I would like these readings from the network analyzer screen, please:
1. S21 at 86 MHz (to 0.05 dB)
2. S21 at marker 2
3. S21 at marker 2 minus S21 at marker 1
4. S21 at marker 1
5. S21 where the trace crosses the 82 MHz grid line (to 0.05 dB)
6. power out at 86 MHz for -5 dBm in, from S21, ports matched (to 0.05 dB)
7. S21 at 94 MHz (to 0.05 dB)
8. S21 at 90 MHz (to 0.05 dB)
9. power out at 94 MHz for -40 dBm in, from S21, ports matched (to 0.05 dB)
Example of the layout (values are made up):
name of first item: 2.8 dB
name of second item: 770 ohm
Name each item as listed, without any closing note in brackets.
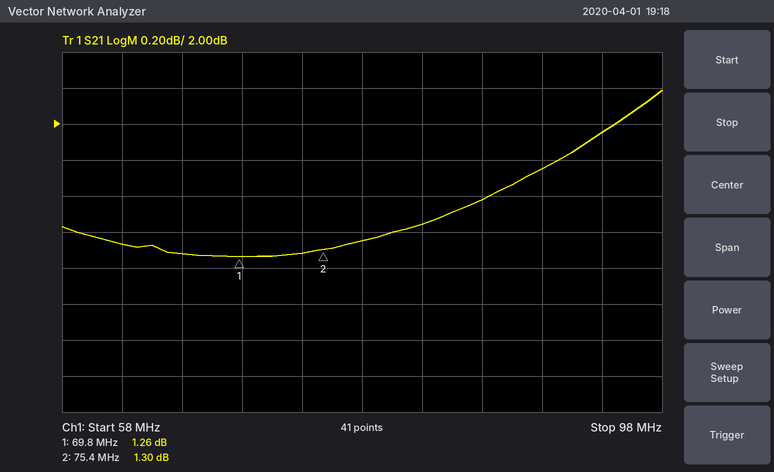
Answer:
S21 at 86 MHz: 1.60 dB
S21 at marker 2: 1.30 dB
S21 at marker 2 minus S21 at marker 1: 0.04 dB
S21 at marker 1: 1.26 dB
S21 where the trace crosses the 82 MHz grid line: 1.45 dB
power out at 86 MHz for -5 dBm in, from S21, ports matched: -3.40 dBm
S21 at 94 MHz: 1.95 dB
S21 at 90 MHz: 1.75 dB
power out at 94 MHz for -40 dBm in, from S21, ports matched: -38.05 dBm
